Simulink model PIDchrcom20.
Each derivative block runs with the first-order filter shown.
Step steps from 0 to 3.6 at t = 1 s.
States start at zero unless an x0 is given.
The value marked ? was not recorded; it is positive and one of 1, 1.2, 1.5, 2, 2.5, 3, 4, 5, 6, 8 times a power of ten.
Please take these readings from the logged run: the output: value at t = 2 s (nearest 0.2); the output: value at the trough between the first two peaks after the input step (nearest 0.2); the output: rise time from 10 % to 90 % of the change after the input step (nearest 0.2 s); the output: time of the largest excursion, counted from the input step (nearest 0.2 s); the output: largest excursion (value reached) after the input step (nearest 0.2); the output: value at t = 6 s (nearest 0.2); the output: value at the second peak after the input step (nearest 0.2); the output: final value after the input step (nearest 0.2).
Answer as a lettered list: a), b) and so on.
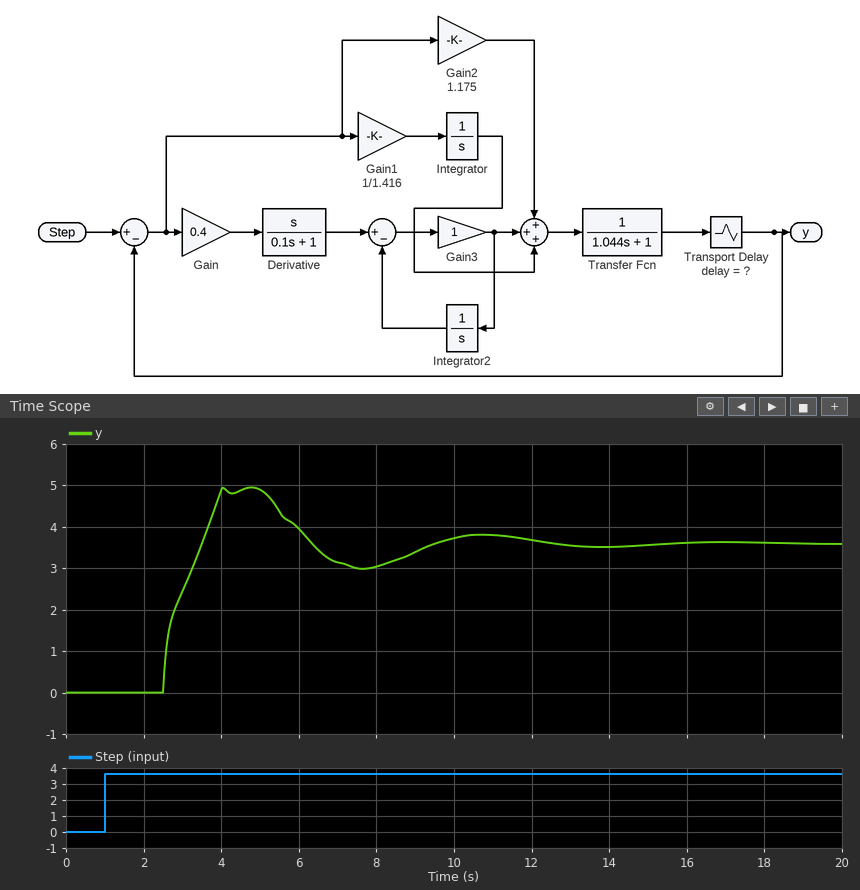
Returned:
a) 0.0
b) 3.0
c) 0.8 s
d) 3.8 s
e) 5.0
f) 4.0
g) 3.8
h) 3.6
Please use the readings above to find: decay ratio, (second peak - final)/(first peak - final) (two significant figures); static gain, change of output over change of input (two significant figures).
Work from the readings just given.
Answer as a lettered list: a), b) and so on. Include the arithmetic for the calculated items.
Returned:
a) (3.8 - 3.6) / (5 - 3.6) = 0.14
b) (3.6 - 0) / (3.6 - 0) = 1.0
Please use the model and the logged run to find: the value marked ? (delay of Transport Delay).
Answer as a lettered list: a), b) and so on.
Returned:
a) 1.5
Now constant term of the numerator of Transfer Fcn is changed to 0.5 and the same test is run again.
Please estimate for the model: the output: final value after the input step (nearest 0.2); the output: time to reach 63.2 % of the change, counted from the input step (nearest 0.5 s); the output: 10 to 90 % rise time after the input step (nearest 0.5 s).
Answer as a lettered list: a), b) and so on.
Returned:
a) 3.6
b) 3.0 s
c) 2.5 s
